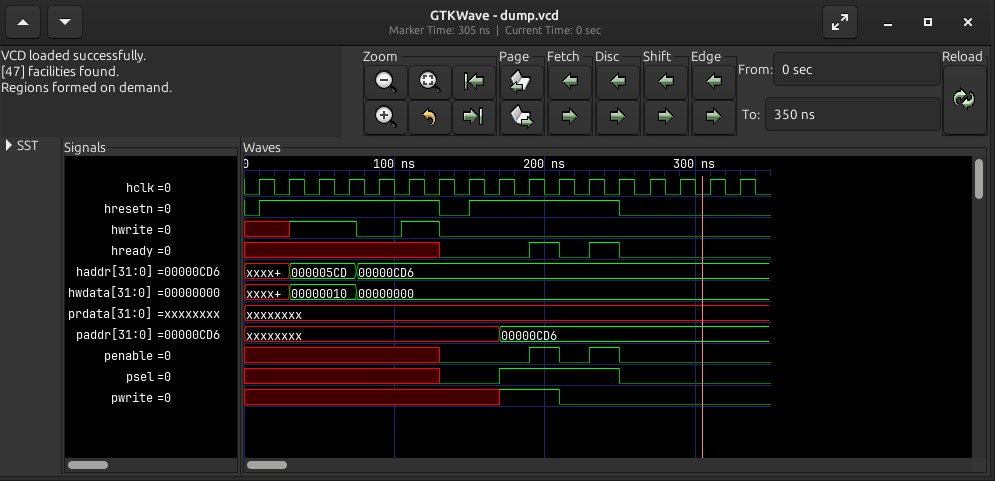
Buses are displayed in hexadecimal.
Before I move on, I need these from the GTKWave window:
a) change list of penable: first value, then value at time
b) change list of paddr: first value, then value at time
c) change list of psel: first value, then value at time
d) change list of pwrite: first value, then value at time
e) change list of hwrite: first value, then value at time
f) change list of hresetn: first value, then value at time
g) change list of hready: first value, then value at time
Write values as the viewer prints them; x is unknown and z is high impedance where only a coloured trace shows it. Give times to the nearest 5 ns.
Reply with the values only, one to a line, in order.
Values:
x, 0 at 130 ns, 1 at 190 ns, 0 at 210 ns, 1 at 230 ns, 0 at 250 ns
xxxxxxxx, 00000CD6 at 170 ns
x, 0 at 130 ns, 1 at 170 ns, 0 at 250 ns
x, 1 at 170 ns, 0 at 210 ns
x, 1 at 30 ns, 0 at 75 ns, 1 at 105 ns, 0 at 130 ns
0, 1 at 10 ns, 0 at 130 ns, 1 at 150 ns, 0 at 250 ns
x, 0 at 130 ns, 1 at 190 ns, 0 at 210 ns, 1 at 230 ns, 0 at 250 ns
